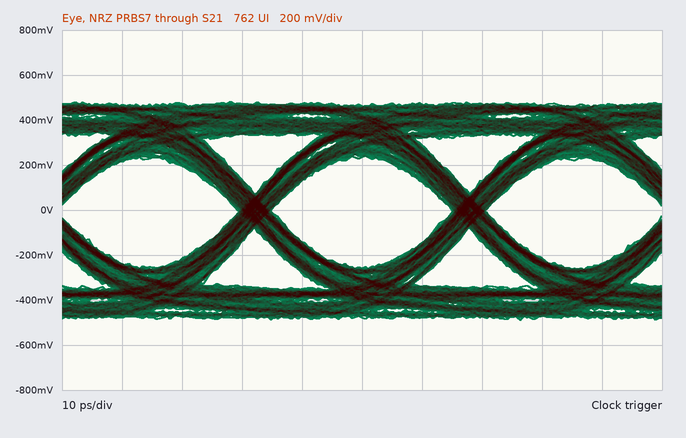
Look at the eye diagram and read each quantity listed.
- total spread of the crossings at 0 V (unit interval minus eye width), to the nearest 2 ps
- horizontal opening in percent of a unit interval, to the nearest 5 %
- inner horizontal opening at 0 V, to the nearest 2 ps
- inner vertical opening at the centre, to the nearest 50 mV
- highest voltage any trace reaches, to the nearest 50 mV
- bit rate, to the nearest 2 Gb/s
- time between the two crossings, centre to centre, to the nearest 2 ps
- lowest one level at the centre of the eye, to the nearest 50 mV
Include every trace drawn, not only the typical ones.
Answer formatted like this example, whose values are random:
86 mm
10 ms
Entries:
6 ps
85 %
30 ps
500 mV
500 mV
28 Gb/s
36 ps
250 mV
